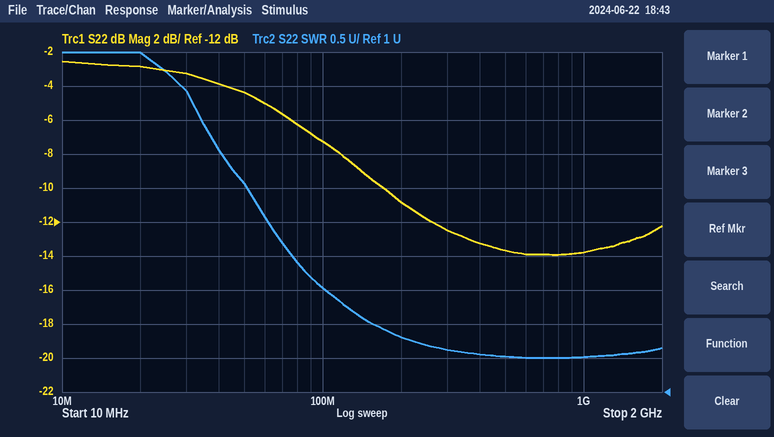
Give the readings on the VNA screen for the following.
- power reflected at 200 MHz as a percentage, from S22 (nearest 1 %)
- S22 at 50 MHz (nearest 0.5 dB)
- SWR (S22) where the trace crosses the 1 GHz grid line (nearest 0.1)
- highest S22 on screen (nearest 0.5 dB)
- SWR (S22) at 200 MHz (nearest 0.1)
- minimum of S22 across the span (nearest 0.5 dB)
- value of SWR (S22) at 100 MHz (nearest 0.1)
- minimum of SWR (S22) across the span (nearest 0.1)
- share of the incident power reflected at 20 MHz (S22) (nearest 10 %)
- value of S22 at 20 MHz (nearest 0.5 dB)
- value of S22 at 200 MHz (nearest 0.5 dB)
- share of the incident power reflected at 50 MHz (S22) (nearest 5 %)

8 %
-4.5 dB
1.5
-2.5 dB
1.8
-14.0 dB
2.5
1.5
50 %
-3.0 dB
-11.0 dB
35 %
